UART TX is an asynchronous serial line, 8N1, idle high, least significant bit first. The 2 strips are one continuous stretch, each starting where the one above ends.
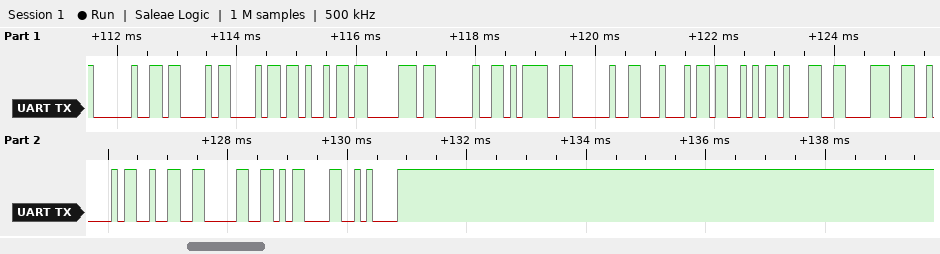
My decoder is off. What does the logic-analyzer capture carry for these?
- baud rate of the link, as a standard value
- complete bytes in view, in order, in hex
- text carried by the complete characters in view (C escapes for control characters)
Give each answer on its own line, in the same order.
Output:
9600 baud
20 43 68 69 70 20 3D 20 44 53 31 38 42 32 30 0D 0A
" Chip = DS18B20\r\n"
